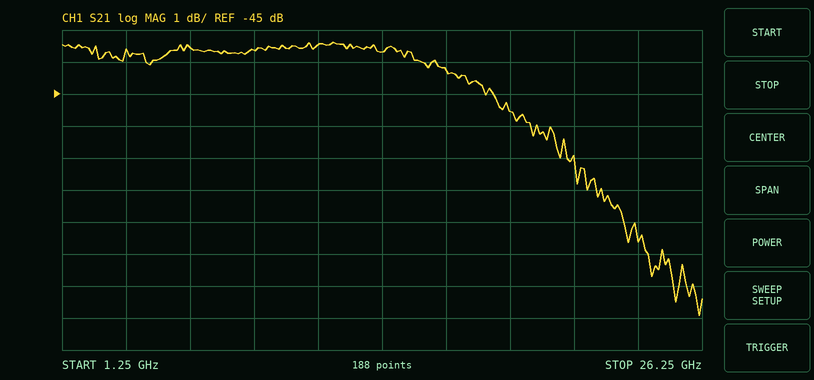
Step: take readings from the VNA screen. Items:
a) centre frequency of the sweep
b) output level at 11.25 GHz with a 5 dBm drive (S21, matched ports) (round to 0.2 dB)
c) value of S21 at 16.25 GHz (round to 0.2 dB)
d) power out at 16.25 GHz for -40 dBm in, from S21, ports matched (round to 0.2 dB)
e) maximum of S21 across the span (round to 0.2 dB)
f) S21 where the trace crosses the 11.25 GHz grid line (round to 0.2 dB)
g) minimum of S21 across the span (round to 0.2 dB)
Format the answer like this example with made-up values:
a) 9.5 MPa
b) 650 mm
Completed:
a) 13.75 GHz
b) -38.4 dBm
c) -44.2 dB
d) -84.2 dBm
e) -43.4 dB
f) -43.4 dB
g) -52.0 dB
